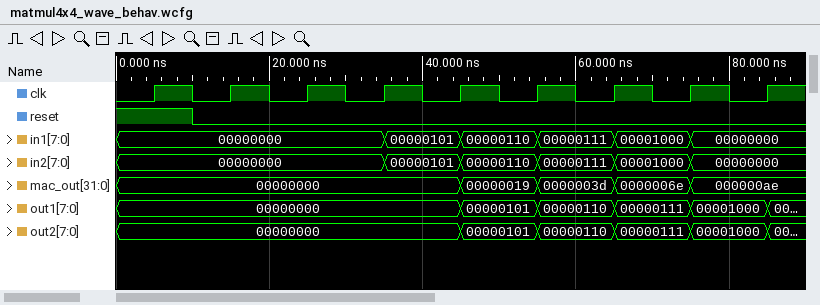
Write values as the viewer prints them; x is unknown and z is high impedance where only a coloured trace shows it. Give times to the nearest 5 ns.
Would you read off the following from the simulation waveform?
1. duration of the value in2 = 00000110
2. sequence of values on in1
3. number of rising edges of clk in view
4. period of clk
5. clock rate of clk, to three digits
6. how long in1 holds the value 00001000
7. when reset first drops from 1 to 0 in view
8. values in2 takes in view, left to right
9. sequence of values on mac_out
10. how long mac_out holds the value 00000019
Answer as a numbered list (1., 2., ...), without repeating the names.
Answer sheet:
1. 10 ns
2. 00000000, 00000101, 00000110, 00000111, 00001000, 00000000
3. 9
4. 10 ns
5. 100 MHz
6. 10 ns
7. 10 ns
8. 00000000, 00000101, 00000110, 00000111, 00001000, 00000000
9. 00000000, 00000019, 0000003d, 0000006e, 000000ae
10. 10 ns
